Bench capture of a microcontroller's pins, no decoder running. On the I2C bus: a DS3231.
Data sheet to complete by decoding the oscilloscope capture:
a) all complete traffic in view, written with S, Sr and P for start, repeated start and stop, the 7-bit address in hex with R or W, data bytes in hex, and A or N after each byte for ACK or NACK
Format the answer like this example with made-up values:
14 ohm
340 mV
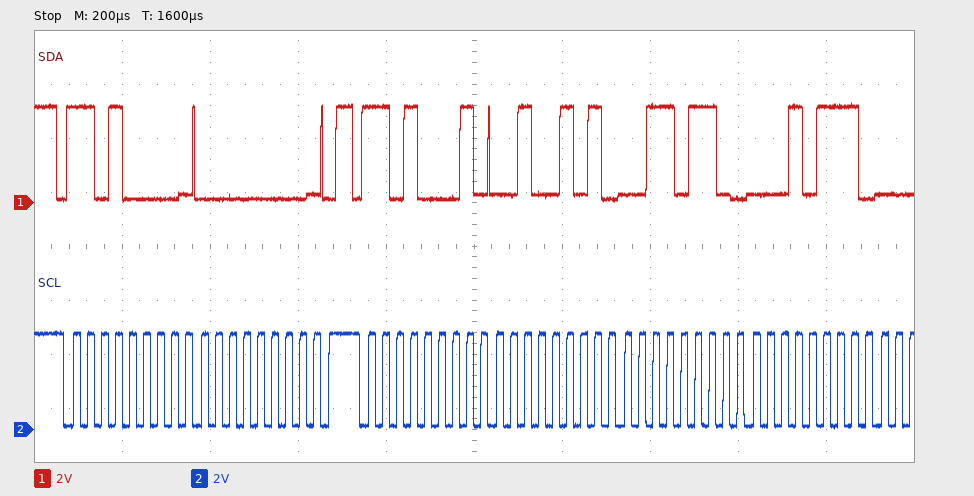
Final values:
S 68W A 00 A P S 68R A 25 A 36 A 17 A
